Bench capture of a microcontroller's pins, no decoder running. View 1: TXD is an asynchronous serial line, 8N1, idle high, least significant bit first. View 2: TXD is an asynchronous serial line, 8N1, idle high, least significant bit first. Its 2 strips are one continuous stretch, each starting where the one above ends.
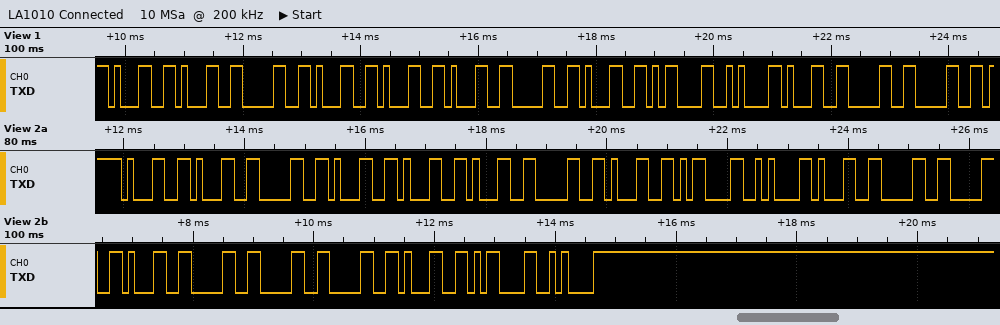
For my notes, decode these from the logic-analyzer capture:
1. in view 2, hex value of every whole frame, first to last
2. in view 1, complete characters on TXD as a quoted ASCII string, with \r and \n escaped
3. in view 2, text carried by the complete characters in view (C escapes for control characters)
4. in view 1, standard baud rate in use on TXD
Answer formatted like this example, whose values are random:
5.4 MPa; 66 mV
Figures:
31 31 30 31 31 31 30 31 0D 0A 31 30 30 31 30 30 30 31 0D 0A; "11011101\r\n100"; "11011101\r\n10010001\r\n"; 9600 baud
